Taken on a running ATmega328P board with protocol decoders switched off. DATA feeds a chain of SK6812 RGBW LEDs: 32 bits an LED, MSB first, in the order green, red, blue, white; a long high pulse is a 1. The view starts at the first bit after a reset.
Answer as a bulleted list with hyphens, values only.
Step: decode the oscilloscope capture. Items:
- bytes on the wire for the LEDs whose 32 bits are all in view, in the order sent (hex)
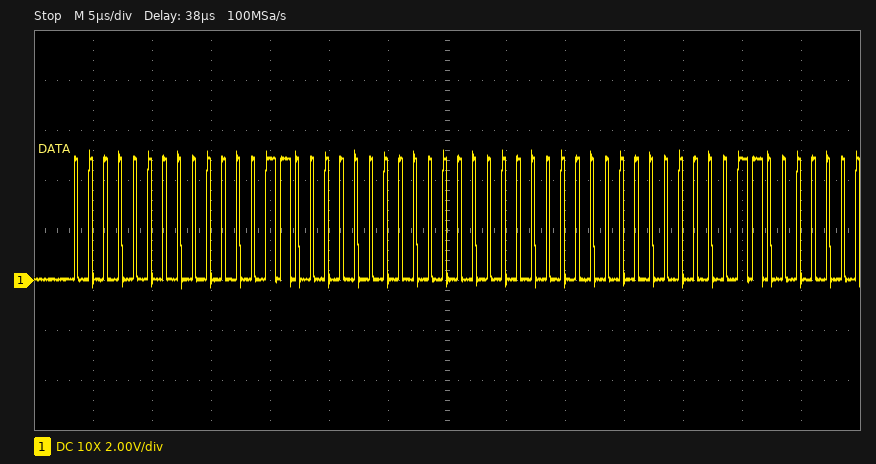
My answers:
- 00 06 00 00
